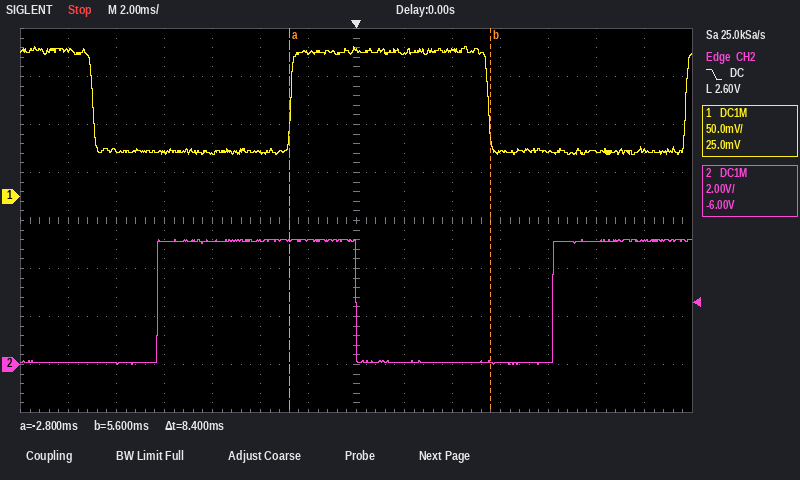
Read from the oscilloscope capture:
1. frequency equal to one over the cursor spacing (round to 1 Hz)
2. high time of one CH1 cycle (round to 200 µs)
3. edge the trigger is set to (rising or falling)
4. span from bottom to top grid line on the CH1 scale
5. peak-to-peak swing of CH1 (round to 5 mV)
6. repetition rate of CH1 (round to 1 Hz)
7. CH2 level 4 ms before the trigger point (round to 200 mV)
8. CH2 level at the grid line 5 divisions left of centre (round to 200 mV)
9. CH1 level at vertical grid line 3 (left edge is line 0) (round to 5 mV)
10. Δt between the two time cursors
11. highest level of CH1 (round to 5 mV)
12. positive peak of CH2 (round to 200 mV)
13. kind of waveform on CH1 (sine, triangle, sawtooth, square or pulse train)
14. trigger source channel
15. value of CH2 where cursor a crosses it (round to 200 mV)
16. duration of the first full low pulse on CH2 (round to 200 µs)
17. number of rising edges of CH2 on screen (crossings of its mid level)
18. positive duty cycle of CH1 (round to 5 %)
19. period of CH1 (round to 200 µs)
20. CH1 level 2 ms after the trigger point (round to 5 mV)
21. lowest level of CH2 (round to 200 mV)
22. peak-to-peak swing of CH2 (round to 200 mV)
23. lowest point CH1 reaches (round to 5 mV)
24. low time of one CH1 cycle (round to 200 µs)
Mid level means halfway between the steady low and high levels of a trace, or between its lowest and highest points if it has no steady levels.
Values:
119 Hz
8.2 ms
falling
400 mV
110 mV
61 Hz
5.2 V
0.0 V
45 mV
8.4 ms
155 mV
5.2 V
square
CH2
5.2 V
8.2 ms
2
50 %
16.4 ms
150 mV
0.0 V
5.2 V
45 mV
8.2 ms
